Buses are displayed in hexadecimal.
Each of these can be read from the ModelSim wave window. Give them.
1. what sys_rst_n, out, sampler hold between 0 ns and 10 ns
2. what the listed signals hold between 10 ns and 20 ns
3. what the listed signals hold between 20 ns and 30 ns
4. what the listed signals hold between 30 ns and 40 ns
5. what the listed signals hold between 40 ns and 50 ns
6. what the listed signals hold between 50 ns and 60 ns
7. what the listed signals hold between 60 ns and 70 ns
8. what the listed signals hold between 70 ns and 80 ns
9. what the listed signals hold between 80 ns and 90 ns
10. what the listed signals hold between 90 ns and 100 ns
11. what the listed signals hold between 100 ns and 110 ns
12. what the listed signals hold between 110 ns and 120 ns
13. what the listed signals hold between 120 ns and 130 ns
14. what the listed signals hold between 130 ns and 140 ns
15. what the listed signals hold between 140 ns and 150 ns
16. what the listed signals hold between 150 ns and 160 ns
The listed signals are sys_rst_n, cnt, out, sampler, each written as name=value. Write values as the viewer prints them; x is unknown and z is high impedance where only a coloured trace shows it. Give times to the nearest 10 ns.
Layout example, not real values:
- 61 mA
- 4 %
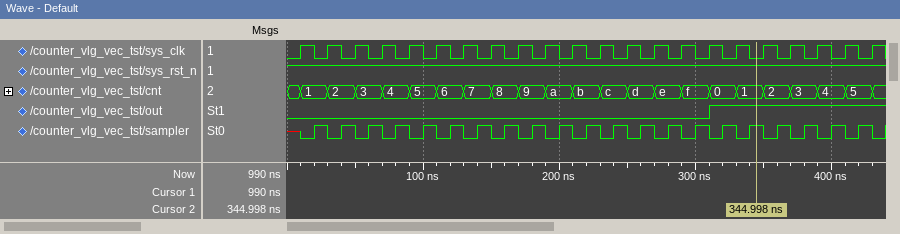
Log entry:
- sys_rst_n=1, out=0, sampler=x
- sys_rst_n=1, cnt=1, out=0, sampler=0
- sys_rst_n=1, cnt=1, out=0, sampler=1
- sys_rst_n=1, cnt=2, out=0, sampler=0
- sys_rst_n=1, cnt=2, out=0, sampler=1
- sys_rst_n=1, cnt=3, out=0, sampler=0
- sys_rst_n=1, cnt=3, out=0, sampler=1
- sys_rst_n=1, cnt=4, out=0, sampler=0
- sys_rst_n=1, cnt=4, out=0, sampler=1
- sys_rst_n=1, cnt=5, out=0, sampler=0
- sys_rst_n=1, cnt=5, out=0, sampler=1
- sys_rst_n=1, cnt=6, out=0, sampler=0
- sys_rst_n=1, cnt=6, out=0, sampler=1
- sys_rst_n=1, cnt=7, out=0, sampler=0
- sys_rst_n=1, cnt=7, out=0, sampler=1
- sys_rst_n=1, cnt=8, out=0, sampler=0
